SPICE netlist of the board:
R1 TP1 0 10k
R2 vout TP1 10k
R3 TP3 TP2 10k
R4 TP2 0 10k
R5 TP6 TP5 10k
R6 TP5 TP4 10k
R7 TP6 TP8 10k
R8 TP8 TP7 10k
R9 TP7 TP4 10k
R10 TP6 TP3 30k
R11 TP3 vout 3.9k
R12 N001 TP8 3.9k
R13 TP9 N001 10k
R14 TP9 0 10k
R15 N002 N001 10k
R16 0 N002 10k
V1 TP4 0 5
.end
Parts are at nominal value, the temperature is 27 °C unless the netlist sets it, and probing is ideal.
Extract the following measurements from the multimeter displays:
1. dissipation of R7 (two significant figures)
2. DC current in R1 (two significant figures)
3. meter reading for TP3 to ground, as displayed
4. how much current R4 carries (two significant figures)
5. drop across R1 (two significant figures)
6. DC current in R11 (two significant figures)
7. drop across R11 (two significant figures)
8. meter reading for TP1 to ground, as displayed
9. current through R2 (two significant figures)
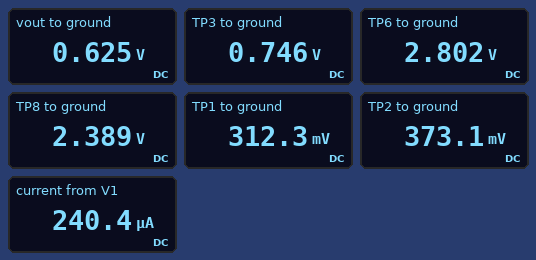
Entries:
17 µW
31 µA
0.746 V
37 µA
310 mV
31 µA
120 mV
312.3 mV
31 µA
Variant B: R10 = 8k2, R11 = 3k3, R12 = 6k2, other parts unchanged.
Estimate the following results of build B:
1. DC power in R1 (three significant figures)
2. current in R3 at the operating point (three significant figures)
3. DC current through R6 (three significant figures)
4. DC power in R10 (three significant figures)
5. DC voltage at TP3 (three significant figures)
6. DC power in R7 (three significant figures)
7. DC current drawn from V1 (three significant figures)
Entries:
33.2 µW
67.2 µA
132 µA
128 µW
1.34 V
466 nW
267 µA
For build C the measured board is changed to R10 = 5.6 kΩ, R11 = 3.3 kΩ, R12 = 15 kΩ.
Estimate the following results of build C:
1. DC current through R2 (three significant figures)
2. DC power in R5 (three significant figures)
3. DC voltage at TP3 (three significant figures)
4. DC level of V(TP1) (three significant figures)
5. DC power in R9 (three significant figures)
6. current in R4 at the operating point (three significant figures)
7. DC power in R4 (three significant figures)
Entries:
68.0 µA
168 µW
1.58 V
680 mV
146 µW
79.2 µA
62.7 µW
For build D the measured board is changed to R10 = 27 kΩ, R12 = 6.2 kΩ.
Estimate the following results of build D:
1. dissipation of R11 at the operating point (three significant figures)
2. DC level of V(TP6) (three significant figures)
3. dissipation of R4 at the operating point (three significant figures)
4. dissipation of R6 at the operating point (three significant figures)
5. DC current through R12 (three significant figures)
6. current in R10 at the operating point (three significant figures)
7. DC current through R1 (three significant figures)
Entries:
4.58 µW
2.85 V
16.8 µW
116 µW
156 µA
75.2 µA
34.3 µA
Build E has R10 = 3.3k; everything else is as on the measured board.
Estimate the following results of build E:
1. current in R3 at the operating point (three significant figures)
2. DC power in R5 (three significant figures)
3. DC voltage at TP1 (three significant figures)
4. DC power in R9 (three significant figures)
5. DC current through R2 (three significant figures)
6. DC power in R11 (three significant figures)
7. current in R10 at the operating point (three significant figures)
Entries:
79.3 µA
215 µW
664 mV
216 µW
66.4 µA
17.2 µW
146 µA
